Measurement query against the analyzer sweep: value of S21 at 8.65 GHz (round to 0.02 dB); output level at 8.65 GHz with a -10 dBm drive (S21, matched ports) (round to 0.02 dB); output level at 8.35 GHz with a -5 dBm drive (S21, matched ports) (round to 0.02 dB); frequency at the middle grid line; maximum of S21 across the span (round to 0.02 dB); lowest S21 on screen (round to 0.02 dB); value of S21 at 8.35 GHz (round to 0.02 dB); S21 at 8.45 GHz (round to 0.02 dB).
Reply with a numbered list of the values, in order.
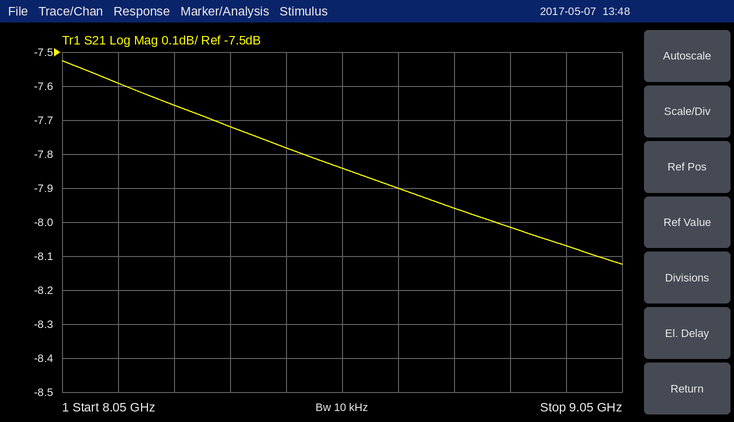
1. -7.90 dB
2. -17.90 dBm
3. -12.72 dBm
4. 8.55 GHz
5. -7.52 dB
6. -8.12 dB
7. -7.72 dB
8. -7.78 dB
